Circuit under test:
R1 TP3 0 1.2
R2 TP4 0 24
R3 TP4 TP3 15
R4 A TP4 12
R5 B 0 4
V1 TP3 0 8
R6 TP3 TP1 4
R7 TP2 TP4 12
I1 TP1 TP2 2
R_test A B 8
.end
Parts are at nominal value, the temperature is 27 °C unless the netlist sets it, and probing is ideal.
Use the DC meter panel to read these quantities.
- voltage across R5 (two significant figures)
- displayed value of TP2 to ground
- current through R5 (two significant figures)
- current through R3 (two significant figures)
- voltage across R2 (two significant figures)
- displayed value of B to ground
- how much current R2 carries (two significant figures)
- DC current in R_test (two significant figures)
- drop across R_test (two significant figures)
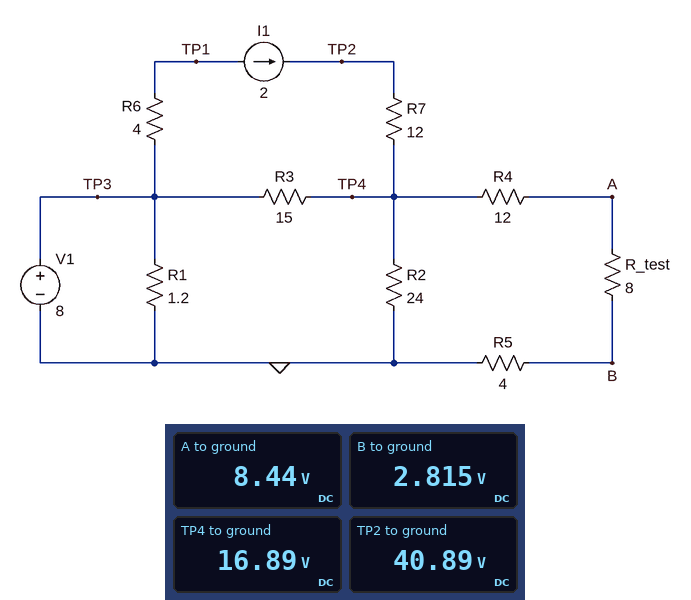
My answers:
2.8 V
40.89 V
700 mA
590 mA
17 V
2.815 V
700 mA
700 mA
5.6 V
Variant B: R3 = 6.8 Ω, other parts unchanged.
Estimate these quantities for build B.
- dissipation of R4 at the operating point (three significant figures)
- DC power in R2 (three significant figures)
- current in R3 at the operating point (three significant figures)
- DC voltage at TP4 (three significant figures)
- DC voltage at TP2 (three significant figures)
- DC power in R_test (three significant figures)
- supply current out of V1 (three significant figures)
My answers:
3.96 W
7.92 W
851 mA
13.8 V
37.8 V
2.64 W
7.82 A
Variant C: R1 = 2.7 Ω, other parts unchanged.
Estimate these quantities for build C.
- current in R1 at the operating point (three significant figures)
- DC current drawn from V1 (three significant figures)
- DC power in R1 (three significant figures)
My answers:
2.96 A
4.37 A
23.7 W
